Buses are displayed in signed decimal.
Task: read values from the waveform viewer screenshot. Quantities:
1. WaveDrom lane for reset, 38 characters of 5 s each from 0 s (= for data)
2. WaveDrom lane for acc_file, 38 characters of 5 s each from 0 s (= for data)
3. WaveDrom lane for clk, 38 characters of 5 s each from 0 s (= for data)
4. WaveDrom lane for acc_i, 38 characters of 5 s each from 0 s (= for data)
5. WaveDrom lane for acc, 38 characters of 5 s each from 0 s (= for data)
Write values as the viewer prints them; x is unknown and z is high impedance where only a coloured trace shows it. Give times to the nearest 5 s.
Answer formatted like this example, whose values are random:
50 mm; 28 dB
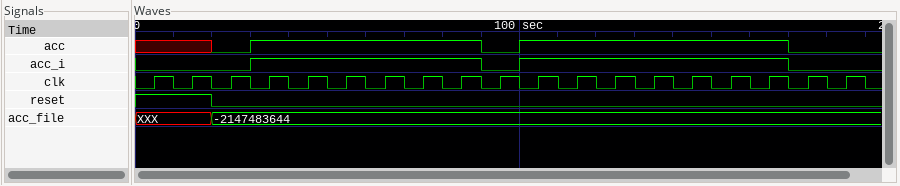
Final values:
{name: 'reset', wave: '1...0.................................'}; {name: 'acc_file', wave: 'x...=.................................', data: '-2147483644'}; {name: 'clk', wave: '01010101010101010101010101010101010101'}; {name: 'acc_i', wave: '0.....1...........0.1.............0...'}; {name: 'acc', wave: 'x...0.1...........0.1.............0...'}
